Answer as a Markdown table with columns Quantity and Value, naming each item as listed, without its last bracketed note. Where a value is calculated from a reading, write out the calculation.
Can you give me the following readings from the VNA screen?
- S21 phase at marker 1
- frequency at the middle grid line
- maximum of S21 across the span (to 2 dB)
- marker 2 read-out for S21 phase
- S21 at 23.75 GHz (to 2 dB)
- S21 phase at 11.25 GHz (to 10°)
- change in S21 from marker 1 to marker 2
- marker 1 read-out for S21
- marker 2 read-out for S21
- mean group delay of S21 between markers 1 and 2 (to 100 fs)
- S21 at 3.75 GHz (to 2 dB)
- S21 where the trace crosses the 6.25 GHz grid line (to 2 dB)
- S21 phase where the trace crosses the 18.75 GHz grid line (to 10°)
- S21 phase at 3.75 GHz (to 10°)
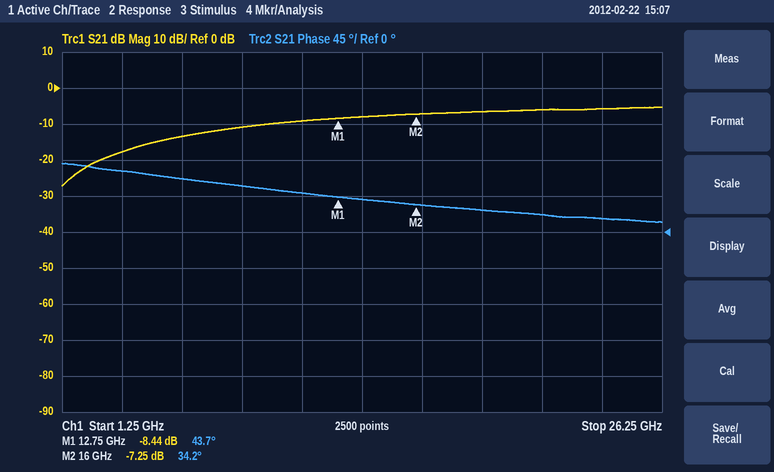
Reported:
| Quantity | Value |
|---|---|
| S21 phase at marker 1 | 43.7° |
| frequency at the middle grid line | 13.75 GHz |
| maximum of S21 across the span | -6 dB |
| marker 2 read-out for S21 phase | 34.2° |
| S21 at 23.75 GHz | -6 dB |
| S21 phase at 11.25 GHz | 50° |
| change in S21 from marker 1 to marker 2 | -7.25 − (-8.44) = 1.19 dB |
| marker 1 read-out for S21 | -8.44 dB |
| marker 2 read-out for S21 | -7.25 dB |
| mean group delay of S21 between markers 1 and 2 | −(34.2° − (43.7°))/(360° × 3.25 GHz) ≈ 8.1 ps |
| S21 at 3.75 GHz | -18 dB |
| S21 where the trace crosses the 6.25 GHz grid line | -14 dB |
| S21 phase where the trace crosses the 18.75 GHz grid line | 30° |
| S21 phase at 3.75 GHz | 80° |
